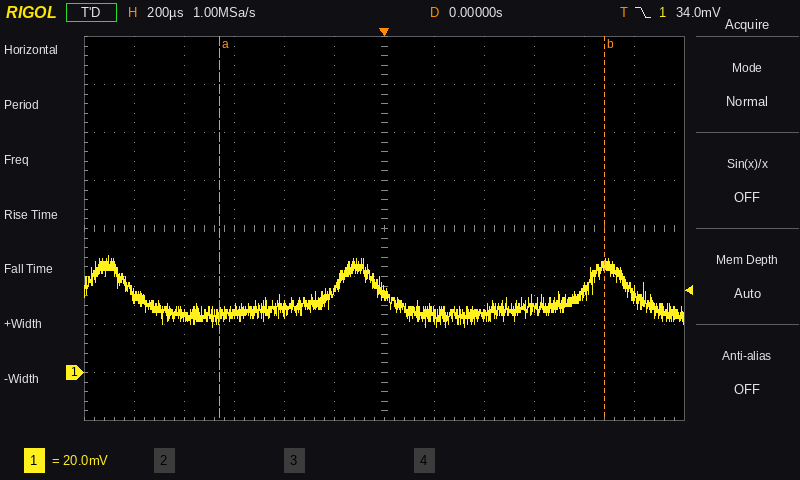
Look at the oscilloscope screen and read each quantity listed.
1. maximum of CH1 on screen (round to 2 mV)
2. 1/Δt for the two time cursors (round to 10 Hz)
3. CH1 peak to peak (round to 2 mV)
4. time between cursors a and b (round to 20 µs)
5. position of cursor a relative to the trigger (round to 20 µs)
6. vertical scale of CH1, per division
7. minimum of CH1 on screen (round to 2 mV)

48 mV
650 Hz
30 mV
1.54 ms
-660 µs
20 mV
18 mV
